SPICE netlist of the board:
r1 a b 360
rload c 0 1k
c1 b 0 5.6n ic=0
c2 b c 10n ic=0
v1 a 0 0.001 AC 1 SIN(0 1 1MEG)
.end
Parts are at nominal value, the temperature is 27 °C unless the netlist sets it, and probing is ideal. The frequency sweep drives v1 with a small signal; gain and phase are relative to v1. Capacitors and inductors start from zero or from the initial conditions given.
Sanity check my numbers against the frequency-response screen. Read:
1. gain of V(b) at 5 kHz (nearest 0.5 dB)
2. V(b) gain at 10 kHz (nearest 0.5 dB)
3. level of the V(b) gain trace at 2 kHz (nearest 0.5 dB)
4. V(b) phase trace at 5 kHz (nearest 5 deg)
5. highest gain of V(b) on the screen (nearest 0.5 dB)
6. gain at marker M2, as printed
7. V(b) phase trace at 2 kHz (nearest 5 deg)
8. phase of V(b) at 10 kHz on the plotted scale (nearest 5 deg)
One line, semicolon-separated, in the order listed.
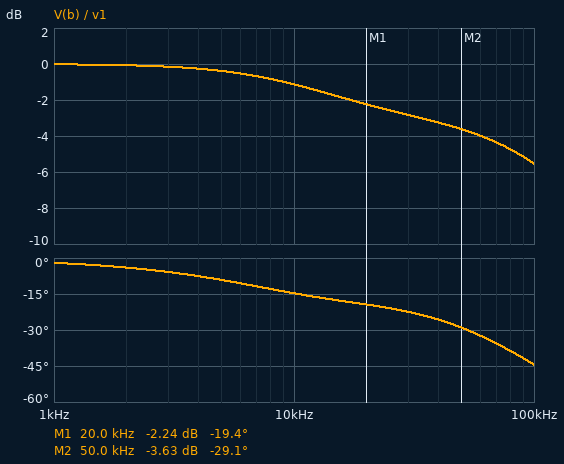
-0.5 dB; -1.0 dB; 0 dB; -10 deg; 0 dB; -3.63 dB; -5 deg; -15 deg
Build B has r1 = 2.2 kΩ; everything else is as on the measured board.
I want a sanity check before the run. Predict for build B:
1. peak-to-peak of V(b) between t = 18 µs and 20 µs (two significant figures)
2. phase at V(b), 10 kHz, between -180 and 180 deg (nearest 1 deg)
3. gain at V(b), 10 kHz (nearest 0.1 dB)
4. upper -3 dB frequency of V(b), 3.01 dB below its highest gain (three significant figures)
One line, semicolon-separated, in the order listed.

26 mV; -47 deg; -7.6 dB; 4.07 kHz
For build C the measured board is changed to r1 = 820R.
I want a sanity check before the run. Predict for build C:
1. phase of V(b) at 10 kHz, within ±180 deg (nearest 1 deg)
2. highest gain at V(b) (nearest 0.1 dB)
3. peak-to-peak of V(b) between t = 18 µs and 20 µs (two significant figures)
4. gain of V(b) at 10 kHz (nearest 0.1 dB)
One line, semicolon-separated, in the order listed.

-28 deg; 0 dB; 69 mV; -2.9 dB
